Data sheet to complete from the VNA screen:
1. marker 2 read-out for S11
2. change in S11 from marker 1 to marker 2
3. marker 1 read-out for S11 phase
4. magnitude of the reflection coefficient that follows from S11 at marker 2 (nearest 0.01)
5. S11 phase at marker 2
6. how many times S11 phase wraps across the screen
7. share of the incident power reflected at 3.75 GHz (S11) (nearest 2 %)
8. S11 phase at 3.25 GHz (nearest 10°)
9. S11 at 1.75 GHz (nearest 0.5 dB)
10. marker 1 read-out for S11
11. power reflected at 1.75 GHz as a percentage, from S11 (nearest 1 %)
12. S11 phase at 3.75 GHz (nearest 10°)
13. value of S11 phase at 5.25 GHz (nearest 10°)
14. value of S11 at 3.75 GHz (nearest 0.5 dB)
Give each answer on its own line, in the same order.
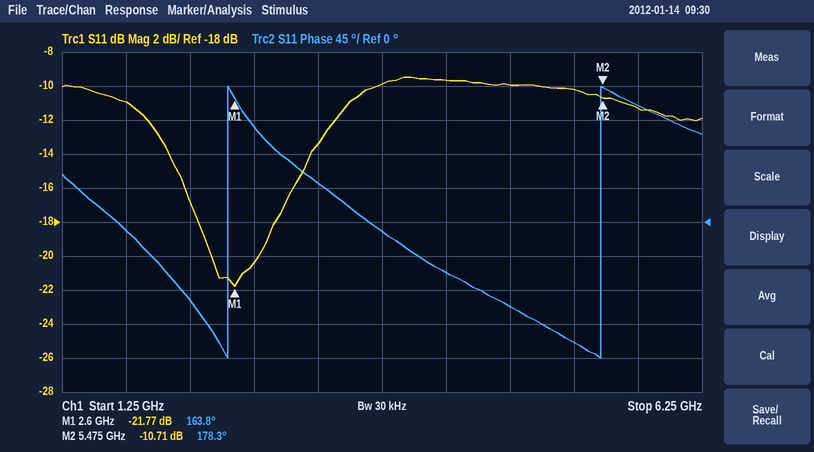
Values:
-10.71 dB
11.06 dB
163.8°
0.29
178.3°
2
10 %
50°
-11.0 dB
-21.77 dB
8 %
-10°
-160°
-10.0 dB
